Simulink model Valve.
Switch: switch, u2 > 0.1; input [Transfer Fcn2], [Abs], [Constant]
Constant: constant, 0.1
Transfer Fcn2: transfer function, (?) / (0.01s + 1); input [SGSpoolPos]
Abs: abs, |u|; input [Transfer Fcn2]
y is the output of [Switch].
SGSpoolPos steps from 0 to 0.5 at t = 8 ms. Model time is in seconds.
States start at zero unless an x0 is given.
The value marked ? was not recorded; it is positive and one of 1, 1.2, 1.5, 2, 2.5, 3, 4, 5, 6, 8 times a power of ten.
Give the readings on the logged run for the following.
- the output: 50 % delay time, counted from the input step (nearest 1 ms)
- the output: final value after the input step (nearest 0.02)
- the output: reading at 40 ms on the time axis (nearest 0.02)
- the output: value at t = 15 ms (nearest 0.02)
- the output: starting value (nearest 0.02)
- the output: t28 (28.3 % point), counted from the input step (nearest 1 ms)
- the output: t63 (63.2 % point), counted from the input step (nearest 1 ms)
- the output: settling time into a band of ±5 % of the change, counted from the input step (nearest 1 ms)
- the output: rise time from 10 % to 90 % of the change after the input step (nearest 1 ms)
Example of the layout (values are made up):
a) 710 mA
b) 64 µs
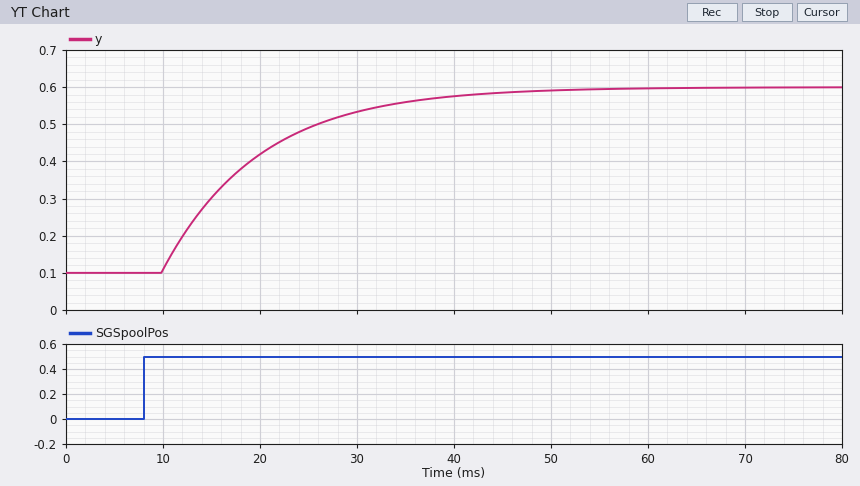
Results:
a) 9 ms
b) 0.60
c) 0.58
d) 0.30
e) 0.10
f) 5 ms
g) 12 ms
h) 32 ms
i) 22 ms
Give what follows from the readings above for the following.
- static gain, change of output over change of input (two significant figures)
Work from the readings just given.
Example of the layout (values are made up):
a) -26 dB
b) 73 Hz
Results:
a) 1.0
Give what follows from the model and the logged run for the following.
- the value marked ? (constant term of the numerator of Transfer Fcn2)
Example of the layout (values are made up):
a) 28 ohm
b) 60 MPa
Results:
a) 1.2
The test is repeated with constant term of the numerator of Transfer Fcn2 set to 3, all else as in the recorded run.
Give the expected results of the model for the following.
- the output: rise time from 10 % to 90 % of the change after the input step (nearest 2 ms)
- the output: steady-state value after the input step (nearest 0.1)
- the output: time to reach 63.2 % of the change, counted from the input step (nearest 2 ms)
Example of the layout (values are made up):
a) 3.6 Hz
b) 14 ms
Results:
a) 22 ms
b) 1.5
c) 10 ms
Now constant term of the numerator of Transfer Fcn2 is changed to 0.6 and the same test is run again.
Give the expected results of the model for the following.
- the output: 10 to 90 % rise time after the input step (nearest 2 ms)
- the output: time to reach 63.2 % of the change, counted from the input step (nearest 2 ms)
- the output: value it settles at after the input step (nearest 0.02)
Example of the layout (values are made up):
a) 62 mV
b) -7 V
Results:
a) 22 ms
b) 14 ms
c) 0.30
